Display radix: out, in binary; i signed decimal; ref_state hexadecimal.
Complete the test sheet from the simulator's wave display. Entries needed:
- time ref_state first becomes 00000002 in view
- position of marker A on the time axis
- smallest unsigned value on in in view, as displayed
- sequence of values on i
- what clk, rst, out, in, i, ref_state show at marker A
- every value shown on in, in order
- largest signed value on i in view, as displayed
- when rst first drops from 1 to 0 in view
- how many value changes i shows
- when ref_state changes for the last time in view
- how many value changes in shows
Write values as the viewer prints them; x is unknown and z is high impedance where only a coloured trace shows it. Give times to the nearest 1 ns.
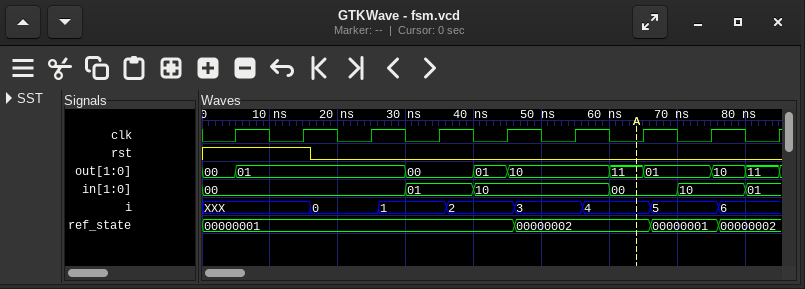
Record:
46 ns
64 ns
00
XXX, 0, 1, 2, 3, 4, 5, 6
clk=0, rst=0, out=11, in=00, i=4, ref_state=00000002
00, 01, 10, 00, 10, 01
6
16 ns
7
76 ns
5
